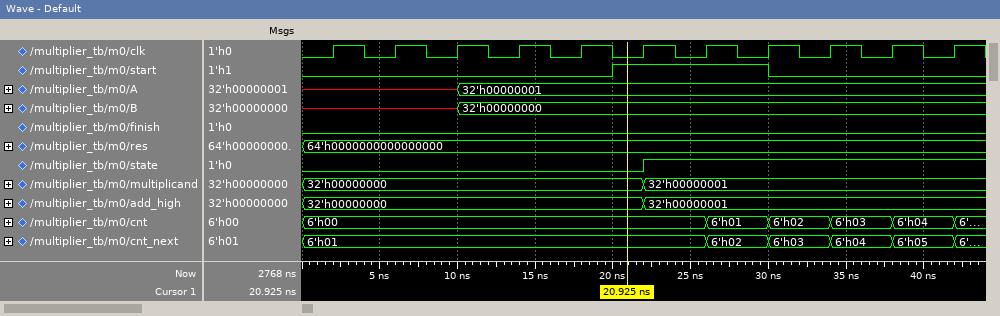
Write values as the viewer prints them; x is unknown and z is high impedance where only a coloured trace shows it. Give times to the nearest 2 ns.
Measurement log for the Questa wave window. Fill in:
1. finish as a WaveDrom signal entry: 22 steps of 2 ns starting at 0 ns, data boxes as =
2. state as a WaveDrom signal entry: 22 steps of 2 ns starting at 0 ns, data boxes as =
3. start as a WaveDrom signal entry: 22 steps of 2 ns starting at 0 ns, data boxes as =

{name: 'finish', wave: '0.....................'}
{name: 'state', wave: '0..........1..........'}
{name: 'start', wave: '0.........1....0......'}
